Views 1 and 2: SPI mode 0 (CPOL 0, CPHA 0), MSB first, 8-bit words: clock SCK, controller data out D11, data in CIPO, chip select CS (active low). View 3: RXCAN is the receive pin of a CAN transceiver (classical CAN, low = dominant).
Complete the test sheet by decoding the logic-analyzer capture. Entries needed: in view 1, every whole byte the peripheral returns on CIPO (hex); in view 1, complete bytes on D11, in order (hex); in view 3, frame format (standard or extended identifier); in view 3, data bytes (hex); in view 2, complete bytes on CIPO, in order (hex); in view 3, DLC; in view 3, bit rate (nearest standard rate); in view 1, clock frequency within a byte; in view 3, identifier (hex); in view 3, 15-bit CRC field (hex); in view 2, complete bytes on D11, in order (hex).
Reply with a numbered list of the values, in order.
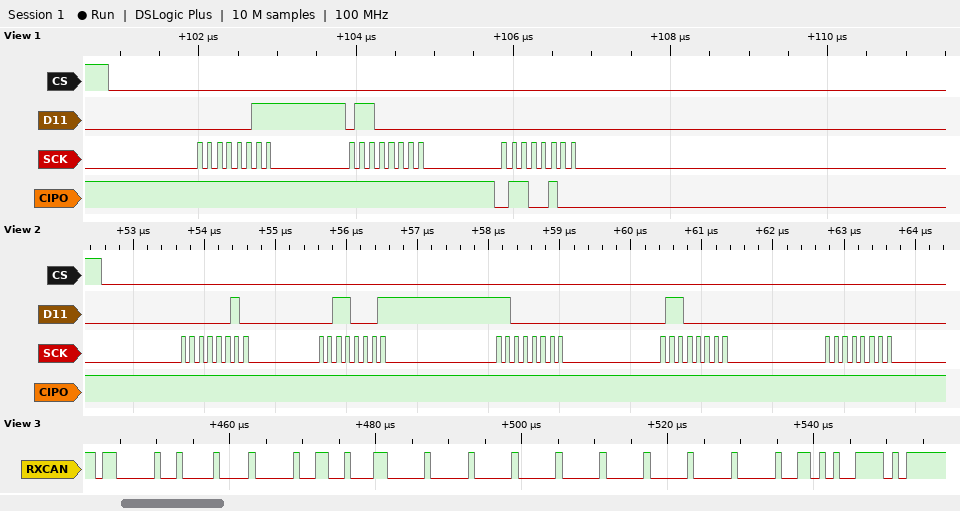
1. 0xFF 0xFF 0x64
2. 0x03 0x60 0x00
3. standard
4. 40 64 60 00 00 00 00 00
5. FF FF FF FF FF
6. 8
7. 1000 kbit/s
8. 8 MHz
9. 0x602
10. 0x1A9E
11. 02 31 C0 60 00
